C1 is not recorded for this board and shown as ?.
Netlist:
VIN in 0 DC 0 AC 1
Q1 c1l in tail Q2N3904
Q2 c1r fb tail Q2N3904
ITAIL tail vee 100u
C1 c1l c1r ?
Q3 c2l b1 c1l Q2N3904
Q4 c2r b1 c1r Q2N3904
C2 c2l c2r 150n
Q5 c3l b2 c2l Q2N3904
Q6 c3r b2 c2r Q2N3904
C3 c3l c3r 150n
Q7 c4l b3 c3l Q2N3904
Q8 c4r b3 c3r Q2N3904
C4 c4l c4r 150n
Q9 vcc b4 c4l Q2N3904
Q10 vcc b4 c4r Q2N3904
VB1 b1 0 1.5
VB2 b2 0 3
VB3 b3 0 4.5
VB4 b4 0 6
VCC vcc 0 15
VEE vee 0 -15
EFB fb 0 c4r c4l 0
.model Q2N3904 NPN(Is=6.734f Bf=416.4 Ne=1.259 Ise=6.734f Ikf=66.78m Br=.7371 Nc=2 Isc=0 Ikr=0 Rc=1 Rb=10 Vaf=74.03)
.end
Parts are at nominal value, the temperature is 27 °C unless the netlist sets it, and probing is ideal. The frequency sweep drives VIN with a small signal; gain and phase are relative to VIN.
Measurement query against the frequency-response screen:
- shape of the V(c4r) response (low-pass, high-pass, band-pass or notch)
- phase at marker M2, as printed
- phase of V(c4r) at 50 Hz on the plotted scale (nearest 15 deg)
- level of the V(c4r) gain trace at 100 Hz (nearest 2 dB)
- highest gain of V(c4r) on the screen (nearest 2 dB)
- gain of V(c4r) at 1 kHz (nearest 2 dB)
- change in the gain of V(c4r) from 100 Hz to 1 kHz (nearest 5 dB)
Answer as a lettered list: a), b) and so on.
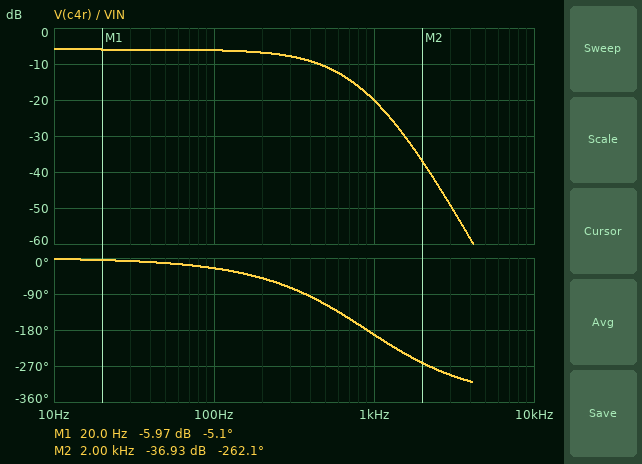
a) low-pass
b) -262.1 deg
c) -15 deg
d) -6 dB
e) -6 dB
f) -20 dB
g) -15 dB
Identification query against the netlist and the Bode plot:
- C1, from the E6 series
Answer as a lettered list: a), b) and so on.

a) 220 nF
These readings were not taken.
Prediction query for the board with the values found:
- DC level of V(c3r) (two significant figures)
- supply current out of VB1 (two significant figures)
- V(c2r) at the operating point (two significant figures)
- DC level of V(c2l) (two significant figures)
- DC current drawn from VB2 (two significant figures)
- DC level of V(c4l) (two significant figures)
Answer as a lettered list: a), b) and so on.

a) 3.9 V
b) 1.1 µA
c) 2.4 V
d) 2.4 V
e) 1.1 µA
f) 5.4 V
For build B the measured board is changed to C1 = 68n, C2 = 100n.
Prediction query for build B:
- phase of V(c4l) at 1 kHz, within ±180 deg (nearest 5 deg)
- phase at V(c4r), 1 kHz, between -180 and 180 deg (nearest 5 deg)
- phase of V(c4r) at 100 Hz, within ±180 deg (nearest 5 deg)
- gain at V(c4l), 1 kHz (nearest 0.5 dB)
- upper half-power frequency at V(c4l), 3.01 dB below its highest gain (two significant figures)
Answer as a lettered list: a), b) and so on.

a) 30 deg
b) -150 deg
c) -20 deg
d) -14.5 dB
e) 530 Hz
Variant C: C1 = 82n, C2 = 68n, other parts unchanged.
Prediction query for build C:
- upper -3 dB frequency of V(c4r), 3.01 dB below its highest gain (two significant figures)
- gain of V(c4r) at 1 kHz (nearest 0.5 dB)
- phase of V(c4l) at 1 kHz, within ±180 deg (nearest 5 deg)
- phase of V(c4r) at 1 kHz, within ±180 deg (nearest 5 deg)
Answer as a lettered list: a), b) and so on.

a) 550 Hz
b) -14.0 dB
c) 35 deg
d) -145 deg
